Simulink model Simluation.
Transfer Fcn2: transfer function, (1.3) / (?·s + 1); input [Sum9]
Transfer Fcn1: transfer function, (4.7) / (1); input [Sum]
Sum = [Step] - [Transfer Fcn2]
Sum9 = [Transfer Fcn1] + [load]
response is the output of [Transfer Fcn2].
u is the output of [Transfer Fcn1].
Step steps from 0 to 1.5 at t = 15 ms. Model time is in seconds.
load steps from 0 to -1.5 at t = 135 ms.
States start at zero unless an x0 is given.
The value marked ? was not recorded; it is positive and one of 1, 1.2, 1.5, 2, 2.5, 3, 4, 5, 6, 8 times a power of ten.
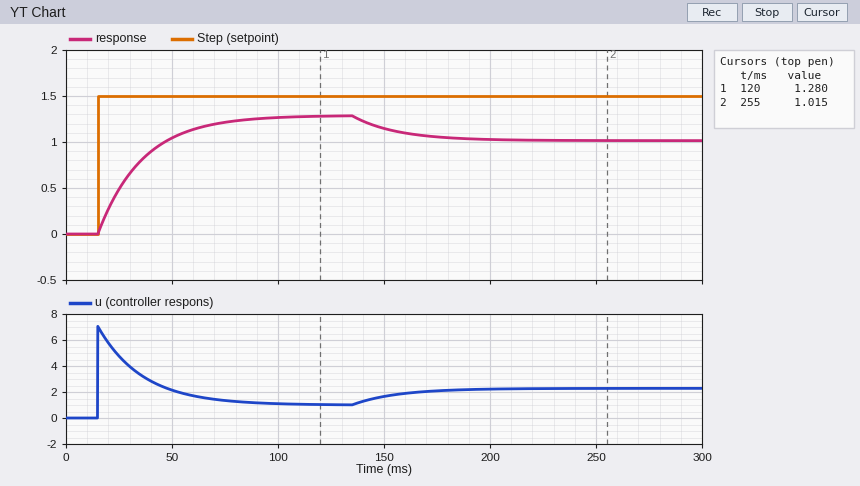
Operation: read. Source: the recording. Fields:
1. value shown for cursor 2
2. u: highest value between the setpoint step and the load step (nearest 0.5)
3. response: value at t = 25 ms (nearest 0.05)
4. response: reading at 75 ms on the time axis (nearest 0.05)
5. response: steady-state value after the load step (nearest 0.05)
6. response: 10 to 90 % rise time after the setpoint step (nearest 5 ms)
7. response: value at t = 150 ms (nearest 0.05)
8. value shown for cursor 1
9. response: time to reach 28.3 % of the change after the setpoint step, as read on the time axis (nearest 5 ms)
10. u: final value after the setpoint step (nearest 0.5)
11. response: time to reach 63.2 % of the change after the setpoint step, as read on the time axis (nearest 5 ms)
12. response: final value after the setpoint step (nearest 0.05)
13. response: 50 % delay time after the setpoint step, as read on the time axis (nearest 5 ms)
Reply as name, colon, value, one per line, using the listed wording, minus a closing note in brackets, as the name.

value shown for cursor 2: 1.015
u: highest value between the setpoint step and the load step: 7.0
response: value at t = 25 ms: 0.50
response: reading at 75 ms on the time axis: 1.20
response: steady-state value after the load step: 1.00
response: 10 to 90 % rise time after the setpoint step: 45 ms
response: value at t = 150 ms: 1.15
value shown for cursor 1: 1.280
response: time to reach 28.3 % of the change after the setpoint step, as read on the time axis: 20 ms
u: final value after the setpoint step: 1.0
response: time to reach 63.2 % of the change after the setpoint step, as read on the time axis: 35 ms
response: final value after the setpoint step: 1.30
response: 50 % delay time after the setpoint step, as read on the time axis: 30 ms
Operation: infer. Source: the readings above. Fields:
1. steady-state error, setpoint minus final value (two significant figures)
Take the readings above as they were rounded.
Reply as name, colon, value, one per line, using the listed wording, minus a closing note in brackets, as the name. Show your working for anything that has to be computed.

steady-state error, setpoint minus final value: 1.5 - 1.3 = 0.20
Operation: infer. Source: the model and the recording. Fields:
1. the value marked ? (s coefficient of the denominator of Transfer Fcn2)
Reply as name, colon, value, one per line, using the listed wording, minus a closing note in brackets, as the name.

the value marked ?: 0.15
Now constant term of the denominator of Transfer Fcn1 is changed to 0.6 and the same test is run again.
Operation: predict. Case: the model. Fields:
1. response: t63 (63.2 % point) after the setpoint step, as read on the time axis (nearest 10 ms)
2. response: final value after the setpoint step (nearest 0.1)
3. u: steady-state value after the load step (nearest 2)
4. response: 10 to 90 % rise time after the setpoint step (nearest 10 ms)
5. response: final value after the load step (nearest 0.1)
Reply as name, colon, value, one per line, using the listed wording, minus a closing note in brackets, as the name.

response: t63 (63.2 % point) after the setpoint step, as read on the time axis: 30 ms
response: final value after the setpoint step: 1.4
u: steady-state value after the load step: 2
response: 10 to 90 % rise time after the setpoint step: 30 ms
response: final value after the load step: 1.2
